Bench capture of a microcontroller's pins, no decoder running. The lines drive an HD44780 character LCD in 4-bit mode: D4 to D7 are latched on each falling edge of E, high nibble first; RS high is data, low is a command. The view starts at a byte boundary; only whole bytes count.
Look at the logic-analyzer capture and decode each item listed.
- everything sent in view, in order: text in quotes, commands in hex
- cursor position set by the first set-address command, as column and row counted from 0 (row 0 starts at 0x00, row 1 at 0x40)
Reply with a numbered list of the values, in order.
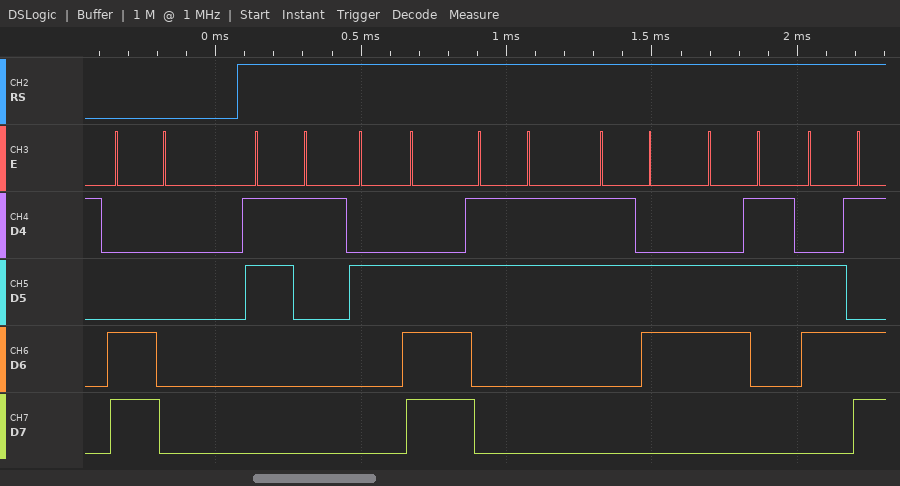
1. 0xC0 "1.36cm"
2. column 0, row 1
